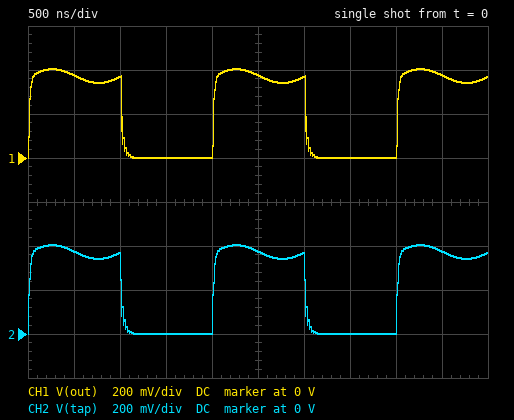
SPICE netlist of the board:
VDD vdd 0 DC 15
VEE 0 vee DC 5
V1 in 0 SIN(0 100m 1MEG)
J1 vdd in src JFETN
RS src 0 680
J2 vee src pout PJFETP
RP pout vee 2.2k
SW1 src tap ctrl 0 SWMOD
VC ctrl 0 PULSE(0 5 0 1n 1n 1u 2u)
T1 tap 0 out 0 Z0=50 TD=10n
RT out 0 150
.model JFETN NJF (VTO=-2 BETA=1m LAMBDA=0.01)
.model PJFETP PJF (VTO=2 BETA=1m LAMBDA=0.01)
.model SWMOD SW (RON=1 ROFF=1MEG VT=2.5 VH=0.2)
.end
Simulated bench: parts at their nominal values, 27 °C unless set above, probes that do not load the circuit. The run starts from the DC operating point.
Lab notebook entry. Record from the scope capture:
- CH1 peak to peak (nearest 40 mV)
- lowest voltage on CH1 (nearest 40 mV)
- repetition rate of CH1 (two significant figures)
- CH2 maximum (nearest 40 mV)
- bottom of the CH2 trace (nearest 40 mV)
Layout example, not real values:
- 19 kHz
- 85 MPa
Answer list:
- 400 mV
- 0 V
- 500 kHz
- 400 mV
- 0 V
